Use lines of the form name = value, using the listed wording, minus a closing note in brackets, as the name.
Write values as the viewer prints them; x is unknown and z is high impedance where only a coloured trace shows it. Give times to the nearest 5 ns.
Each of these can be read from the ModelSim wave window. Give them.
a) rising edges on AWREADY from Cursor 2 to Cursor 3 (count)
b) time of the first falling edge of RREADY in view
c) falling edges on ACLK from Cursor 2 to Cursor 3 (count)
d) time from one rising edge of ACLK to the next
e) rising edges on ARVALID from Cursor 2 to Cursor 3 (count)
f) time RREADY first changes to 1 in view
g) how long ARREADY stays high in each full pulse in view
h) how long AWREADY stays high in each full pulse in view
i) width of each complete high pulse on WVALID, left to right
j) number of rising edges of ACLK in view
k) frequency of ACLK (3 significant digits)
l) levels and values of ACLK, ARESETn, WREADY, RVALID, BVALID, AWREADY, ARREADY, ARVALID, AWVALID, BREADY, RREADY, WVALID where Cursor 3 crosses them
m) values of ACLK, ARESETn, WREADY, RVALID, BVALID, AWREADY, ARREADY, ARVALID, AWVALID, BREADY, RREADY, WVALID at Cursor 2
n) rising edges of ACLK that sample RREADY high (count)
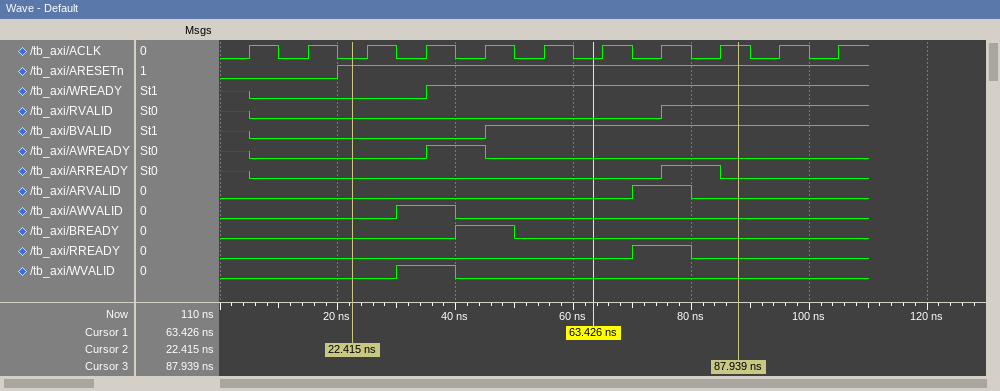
rising edges on AWREADY from Cursor 2 to Cursor 3 = 1
time of the first falling edge of RREADY in view = 80 ns
falling edges on ACLK from Cursor 2 to Cursor 3 = 6
time from one rising edge of ACLK to the next = 10 ns
rising edges on ARVALID from Cursor 2 to Cursor 3 = 1
time RREADY first changes to 1 in view = 70 ns
how long ARREADY stays high in each full pulse in view = 10 ns
how long AWREADY stays high in each full pulse in view = 10 ns
width of each complete high pulse on WVALID, left to right = 10 ns
number of rising edges of ACLK in view = 11
frequency of ACLK = 100 MHz
levels and values of ACLK, ARESETn, WREADY, RVALID, BVALID, AWREADY, ARREADY, ARVALID, AWVALID, BREADY, RREADY, WVALID where Cursor 3 crosses them = ACLK=1, ARESETn=1, WREADY=1, RVALID=1, BVALID=1, AWREADY=0, ARREADY=0, ARVALID=0, AWVALID=0, BREADY=0, RREADY=0, WVALID=0
values of ACLK, ARESETn, WREADY, RVALID, BVALID, AWREADY, ARREADY, ARVALID, AWVALID, BREADY, RREADY, WVALID at Cursor 2 = ACLK=0, ARESETn=1, WREADY=0, RVALID=0, BVALID=0, AWREADY=0, ARREADY=0, ARVALID=0, AWVALID=0, BREADY=0, RREADY=0, WVALID=0
rising edges of ACLK that sample RREADY high = 1
